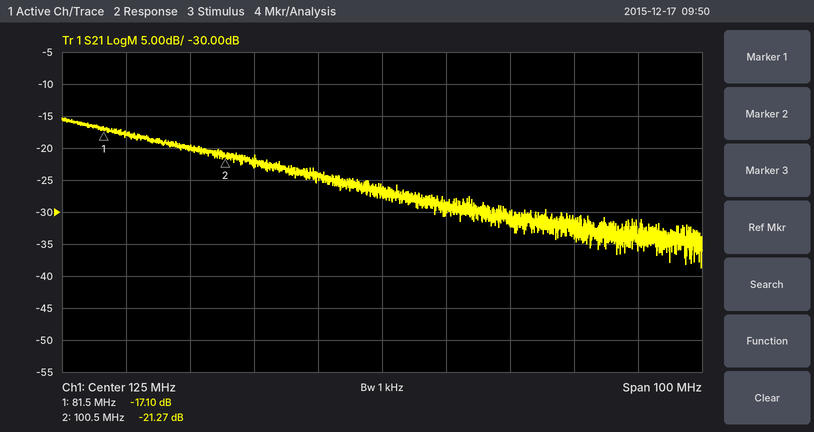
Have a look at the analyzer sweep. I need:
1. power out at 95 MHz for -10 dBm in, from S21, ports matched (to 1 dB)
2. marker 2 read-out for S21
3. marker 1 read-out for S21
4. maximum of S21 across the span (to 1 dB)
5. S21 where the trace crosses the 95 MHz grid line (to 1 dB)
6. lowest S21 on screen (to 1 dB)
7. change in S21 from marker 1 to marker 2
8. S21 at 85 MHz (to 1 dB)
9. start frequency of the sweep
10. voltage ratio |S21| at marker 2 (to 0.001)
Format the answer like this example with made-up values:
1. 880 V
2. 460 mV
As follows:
1. -30 dBm
2. -21.27 dB
3. -17.10 dB
4. -15 dB
5. -20 dB
6. -39 dB
7. -4.17 dB
8. -18 dB
9. 75 MHz
10. 0.086
